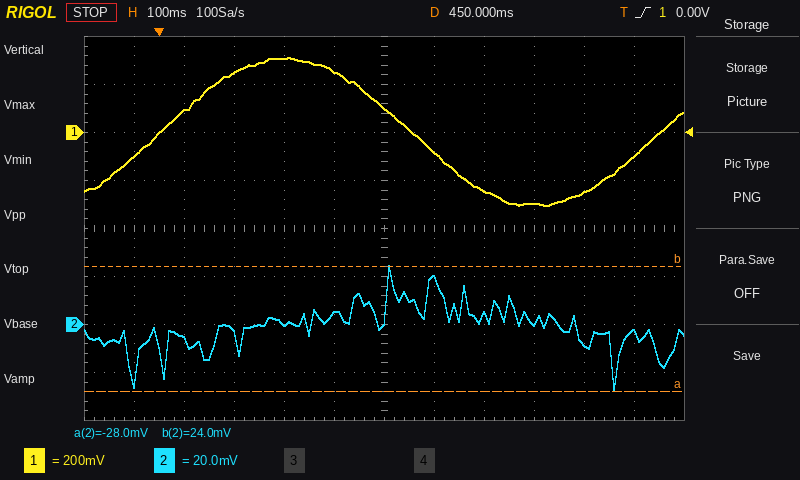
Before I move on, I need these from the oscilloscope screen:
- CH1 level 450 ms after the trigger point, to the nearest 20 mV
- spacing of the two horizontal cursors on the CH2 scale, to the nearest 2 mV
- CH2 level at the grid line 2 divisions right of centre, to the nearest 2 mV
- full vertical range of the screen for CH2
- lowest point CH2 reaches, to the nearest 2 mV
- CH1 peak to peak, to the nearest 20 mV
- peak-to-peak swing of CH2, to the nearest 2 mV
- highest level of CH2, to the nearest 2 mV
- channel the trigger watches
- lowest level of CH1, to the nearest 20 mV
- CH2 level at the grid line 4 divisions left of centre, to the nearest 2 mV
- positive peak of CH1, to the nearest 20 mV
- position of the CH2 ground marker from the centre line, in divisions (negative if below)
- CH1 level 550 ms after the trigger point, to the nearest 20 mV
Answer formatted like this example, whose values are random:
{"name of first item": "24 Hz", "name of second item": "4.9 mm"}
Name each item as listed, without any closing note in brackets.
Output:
{"CH1 level 450 ms after the trigger point, to the nearest 20 mV": "100 mV", "spacing of the two horizontal cursors on the CH2 scale, to the nearest 2 mV": "52 mV", "CH2 level at the grid line 2 divisions right of centre, to the nearest 2 mV": "4 mV", "full vertical range of the screen for CH2": "160 mV", "lowest point CH2 reaches, to the nearest 2 mV": "-28 mV", "CH1 peak to peak, to the nearest 20 mV": "620 mV", "peak-to-peak swing of CH2, to the nearest 2 mV": "52 mV", "highest level of CH2, to the nearest 2 mV": "24 mV", "channel the trigger watches": "CH1", "lowest level of CH1, to the nearest 20 mV": "-300 mV", "CH2 level at the grid line 4 divisions left of centre, to the nearest 2 mV": "-6 mV", "positive peak of CH1, to the nearest 20 mV": "320 mV", "position of the CH2 ground marker from the centre line, in divisions": "-2.0 div", "CH1 level 550 ms after the trigger point, to the nearest 20 mV": "-80 mV"}
